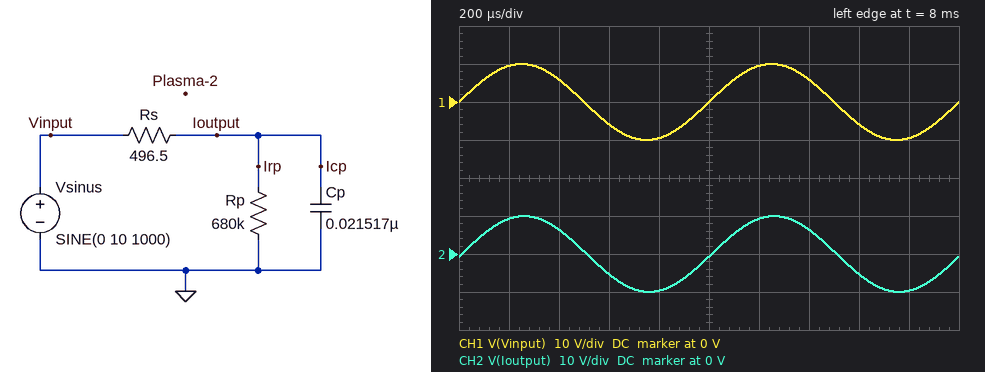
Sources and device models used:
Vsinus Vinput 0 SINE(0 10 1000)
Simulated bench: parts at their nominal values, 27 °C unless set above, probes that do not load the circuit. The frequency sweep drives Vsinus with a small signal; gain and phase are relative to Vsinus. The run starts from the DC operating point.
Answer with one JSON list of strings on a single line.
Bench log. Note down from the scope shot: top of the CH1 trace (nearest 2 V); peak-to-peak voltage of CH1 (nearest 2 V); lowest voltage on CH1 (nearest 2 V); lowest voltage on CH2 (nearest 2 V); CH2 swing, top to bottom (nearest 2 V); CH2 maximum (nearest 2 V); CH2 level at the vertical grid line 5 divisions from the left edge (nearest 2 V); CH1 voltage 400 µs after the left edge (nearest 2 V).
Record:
["10 V", "20 V", "-10 V", "-10 V", "20 V", "10 V", "0 V", "6 V"]
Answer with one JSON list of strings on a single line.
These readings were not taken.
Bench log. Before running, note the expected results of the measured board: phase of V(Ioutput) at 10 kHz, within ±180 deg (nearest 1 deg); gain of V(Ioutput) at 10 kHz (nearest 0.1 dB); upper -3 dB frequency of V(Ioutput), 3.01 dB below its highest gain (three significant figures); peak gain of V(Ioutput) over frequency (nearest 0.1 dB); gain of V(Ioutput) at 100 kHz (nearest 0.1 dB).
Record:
["-34 deg", "-1.6 dB", "14.9 kHz", "0 dB", "-16.6 dB"]
